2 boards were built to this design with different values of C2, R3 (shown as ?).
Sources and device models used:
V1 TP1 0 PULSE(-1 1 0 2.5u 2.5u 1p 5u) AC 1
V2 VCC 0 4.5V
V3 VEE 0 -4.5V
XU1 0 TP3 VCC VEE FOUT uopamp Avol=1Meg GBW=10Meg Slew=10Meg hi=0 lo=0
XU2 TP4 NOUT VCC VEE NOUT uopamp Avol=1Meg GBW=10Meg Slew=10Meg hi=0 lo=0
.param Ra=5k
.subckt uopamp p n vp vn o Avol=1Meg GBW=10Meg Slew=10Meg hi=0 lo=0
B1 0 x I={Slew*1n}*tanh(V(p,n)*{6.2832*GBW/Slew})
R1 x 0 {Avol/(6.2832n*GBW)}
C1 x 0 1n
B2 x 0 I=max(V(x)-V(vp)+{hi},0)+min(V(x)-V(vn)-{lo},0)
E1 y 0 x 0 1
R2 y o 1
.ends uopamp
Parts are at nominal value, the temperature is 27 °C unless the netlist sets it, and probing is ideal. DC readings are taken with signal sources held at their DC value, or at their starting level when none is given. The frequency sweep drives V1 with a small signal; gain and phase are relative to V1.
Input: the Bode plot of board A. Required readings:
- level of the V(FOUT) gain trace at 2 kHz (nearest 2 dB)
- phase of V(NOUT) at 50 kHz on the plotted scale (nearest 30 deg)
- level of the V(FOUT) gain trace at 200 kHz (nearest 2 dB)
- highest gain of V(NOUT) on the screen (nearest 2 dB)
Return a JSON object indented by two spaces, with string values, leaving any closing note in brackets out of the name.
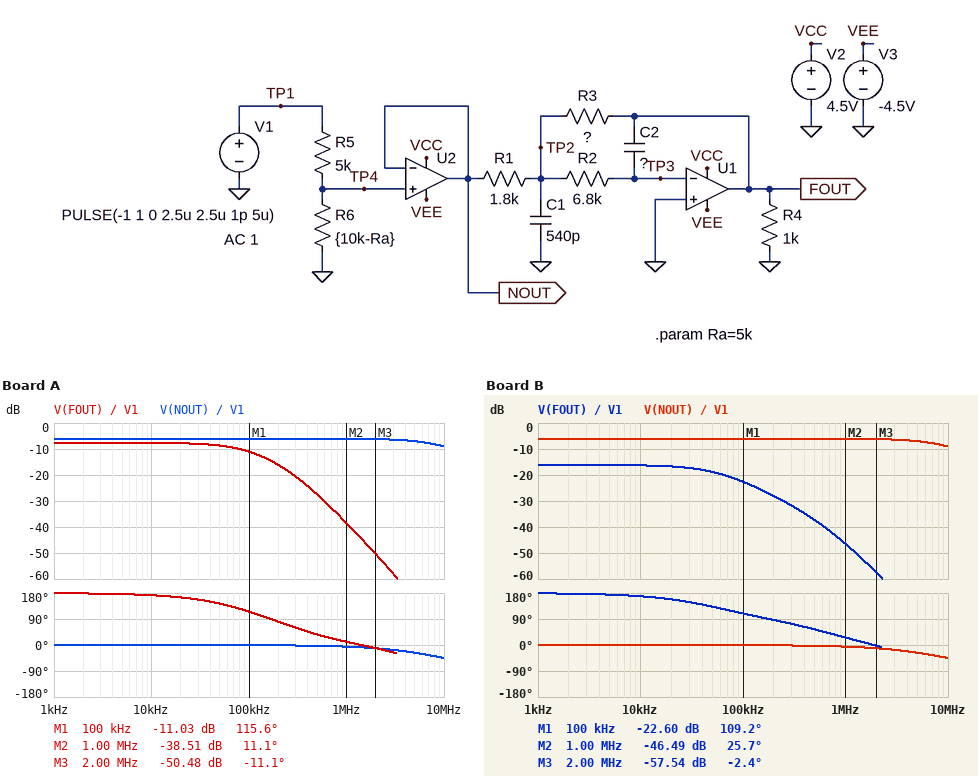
{
  "level of the V(FOUT) gain trace at 2 kHz": "-8 dB",
  "phase of V(NOUT) at 50 kHz on the plotted scale": "0 deg",
  "level of the V(FOUT) gain trace at 200 kHz": "-16 dB",
  "highest gain of V(NOUT) on the screen": "-6 dB"
}
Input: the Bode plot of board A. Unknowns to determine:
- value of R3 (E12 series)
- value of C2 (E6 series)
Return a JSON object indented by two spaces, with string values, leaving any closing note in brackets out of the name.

{
  "value of R3": "1.5 kΩ",
  "value of C2": "150 pF"
}
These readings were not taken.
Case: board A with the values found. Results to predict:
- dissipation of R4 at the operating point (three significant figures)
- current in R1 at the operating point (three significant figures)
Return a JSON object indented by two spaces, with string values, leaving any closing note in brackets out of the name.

{
  "dissipation of R4 at the operating point": "174 µW",
  "current in R1 at the operating point": "278 µA"
}
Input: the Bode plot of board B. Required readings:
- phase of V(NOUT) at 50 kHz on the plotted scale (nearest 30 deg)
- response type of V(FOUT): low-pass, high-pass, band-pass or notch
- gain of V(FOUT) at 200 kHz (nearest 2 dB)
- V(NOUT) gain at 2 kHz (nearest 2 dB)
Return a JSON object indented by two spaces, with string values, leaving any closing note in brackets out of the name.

{
  "phase of V(NOUT) at 50 kHz on the plotted scale": "0 deg",
  "response type of V(FOUT): low-pass, high-pass, band-pass or notch": "low-pass",
  "gain of V(FOUT) at 200 kHz": "-28 dB",
  "V(NOUT) gain at 2 kHz": "-6 dB"
}
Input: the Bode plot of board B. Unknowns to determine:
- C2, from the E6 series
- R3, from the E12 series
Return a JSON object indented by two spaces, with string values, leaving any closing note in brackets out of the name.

{
  "C2, from the E6 series": "330 pF",
  "R3, from the E12 series": "560 Ω"
}
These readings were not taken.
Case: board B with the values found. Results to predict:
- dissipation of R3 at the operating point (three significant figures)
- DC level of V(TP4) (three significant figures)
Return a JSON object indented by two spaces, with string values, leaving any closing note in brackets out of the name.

{
  "dissipation of R3 at the operating point": "43.2 µW",
  "DC level of V(TP4)": "-500 mV"
}
